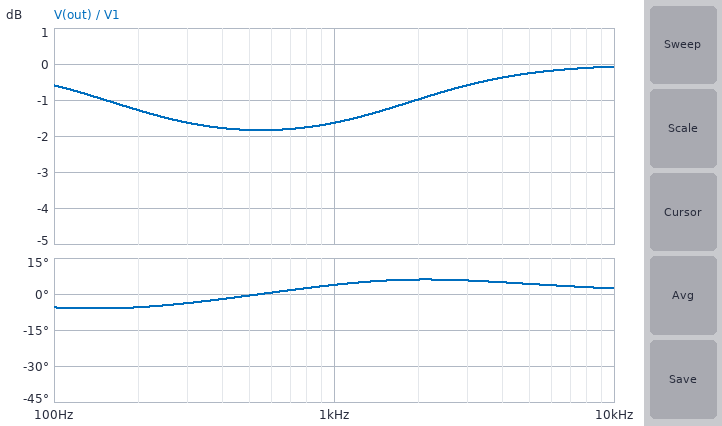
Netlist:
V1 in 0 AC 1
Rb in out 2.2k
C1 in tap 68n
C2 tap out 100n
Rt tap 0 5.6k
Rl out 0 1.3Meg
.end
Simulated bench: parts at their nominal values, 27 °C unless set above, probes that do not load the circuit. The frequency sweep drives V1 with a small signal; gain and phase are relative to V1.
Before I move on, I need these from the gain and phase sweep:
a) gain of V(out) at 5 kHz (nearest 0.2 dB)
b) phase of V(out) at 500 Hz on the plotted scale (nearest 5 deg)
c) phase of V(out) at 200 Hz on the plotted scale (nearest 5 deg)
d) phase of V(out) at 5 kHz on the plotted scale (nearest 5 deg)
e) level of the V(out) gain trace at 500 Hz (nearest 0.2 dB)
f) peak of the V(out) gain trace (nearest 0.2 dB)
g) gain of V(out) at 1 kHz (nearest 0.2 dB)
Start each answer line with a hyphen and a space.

- -0.2 dB
- 0 deg
- -5 deg
- 5 deg
- -1.8 dB
- 0 dB
- -1.6 dB
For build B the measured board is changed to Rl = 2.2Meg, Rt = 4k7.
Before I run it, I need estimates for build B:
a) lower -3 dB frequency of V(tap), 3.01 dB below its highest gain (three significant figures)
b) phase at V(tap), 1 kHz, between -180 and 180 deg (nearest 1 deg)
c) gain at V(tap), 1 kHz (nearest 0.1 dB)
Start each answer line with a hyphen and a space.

- 258 Hz
- 14 deg
- -1.3 dB
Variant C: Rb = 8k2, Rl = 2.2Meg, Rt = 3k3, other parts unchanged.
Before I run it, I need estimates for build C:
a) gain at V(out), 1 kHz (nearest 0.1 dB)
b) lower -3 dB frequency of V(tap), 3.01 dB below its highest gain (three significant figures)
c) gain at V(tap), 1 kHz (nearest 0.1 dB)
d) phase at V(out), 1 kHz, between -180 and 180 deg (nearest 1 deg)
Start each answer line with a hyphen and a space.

- -3.5 dB
- 841 Hz
- -2.4 dB
- 25 deg
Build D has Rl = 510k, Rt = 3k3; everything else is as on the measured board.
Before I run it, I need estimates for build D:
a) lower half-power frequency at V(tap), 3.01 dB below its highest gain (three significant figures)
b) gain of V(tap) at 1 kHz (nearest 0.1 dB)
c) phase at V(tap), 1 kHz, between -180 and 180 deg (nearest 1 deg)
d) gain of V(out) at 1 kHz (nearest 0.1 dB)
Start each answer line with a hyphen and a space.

- 441 Hz
- -1.9 dB
- 18 deg
- -2.8 dB
